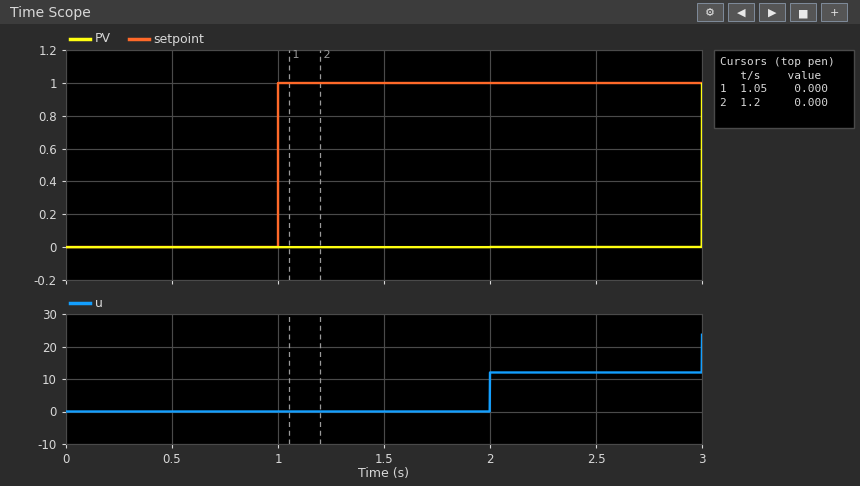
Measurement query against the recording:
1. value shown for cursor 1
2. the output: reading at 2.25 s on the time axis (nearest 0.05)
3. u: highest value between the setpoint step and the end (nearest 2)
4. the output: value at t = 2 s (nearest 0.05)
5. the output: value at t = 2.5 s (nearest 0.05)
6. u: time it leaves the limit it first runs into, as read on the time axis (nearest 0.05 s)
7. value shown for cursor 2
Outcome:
0.000
0.00
12
0.00
0.00
2.00 s
0.000
